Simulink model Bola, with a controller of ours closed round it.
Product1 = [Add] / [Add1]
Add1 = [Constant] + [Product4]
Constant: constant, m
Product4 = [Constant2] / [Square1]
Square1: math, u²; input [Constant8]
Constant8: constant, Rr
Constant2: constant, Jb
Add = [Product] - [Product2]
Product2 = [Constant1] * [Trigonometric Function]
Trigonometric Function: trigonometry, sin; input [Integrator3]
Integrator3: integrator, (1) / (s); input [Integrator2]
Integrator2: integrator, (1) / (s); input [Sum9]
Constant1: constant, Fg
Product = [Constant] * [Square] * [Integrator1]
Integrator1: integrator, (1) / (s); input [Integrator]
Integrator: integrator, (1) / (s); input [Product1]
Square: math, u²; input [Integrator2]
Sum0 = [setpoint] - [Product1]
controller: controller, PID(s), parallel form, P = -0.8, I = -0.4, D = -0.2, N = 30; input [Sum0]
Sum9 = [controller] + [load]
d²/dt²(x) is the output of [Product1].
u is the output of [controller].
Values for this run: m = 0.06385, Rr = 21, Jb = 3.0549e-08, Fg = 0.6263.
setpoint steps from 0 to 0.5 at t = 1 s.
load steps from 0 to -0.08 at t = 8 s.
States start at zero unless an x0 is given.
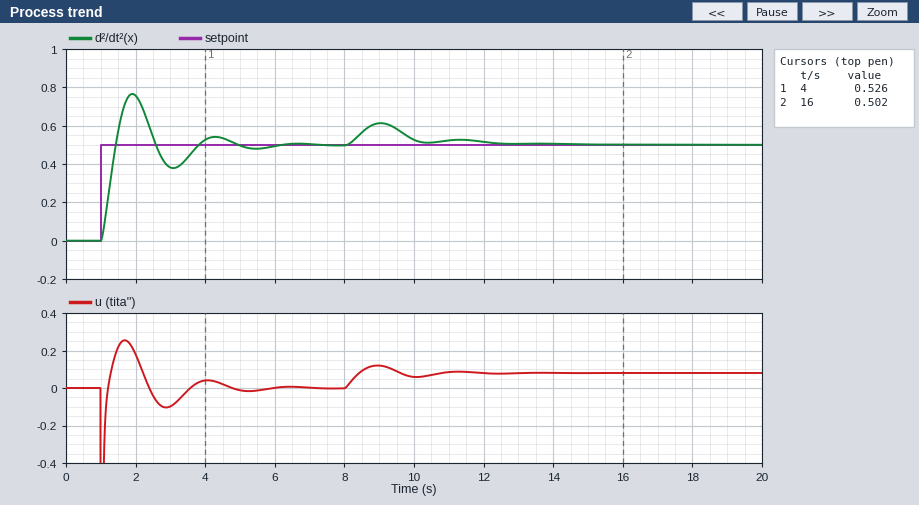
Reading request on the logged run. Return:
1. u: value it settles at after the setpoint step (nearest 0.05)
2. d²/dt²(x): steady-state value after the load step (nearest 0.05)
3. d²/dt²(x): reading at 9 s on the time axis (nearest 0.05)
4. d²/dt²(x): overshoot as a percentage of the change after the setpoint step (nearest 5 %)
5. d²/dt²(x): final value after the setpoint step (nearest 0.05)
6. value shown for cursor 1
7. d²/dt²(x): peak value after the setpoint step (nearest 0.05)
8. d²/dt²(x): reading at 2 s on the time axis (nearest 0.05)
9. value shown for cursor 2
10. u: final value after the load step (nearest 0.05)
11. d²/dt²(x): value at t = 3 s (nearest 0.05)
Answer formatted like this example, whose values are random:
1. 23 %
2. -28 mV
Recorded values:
1. 0.00
2. 0.50
3. 0.60
4. 55 %
5. 0.50
6. 0.526
7. 0.75
8. 0.75
9. 0.502
10. 0.10
11. 0.40
